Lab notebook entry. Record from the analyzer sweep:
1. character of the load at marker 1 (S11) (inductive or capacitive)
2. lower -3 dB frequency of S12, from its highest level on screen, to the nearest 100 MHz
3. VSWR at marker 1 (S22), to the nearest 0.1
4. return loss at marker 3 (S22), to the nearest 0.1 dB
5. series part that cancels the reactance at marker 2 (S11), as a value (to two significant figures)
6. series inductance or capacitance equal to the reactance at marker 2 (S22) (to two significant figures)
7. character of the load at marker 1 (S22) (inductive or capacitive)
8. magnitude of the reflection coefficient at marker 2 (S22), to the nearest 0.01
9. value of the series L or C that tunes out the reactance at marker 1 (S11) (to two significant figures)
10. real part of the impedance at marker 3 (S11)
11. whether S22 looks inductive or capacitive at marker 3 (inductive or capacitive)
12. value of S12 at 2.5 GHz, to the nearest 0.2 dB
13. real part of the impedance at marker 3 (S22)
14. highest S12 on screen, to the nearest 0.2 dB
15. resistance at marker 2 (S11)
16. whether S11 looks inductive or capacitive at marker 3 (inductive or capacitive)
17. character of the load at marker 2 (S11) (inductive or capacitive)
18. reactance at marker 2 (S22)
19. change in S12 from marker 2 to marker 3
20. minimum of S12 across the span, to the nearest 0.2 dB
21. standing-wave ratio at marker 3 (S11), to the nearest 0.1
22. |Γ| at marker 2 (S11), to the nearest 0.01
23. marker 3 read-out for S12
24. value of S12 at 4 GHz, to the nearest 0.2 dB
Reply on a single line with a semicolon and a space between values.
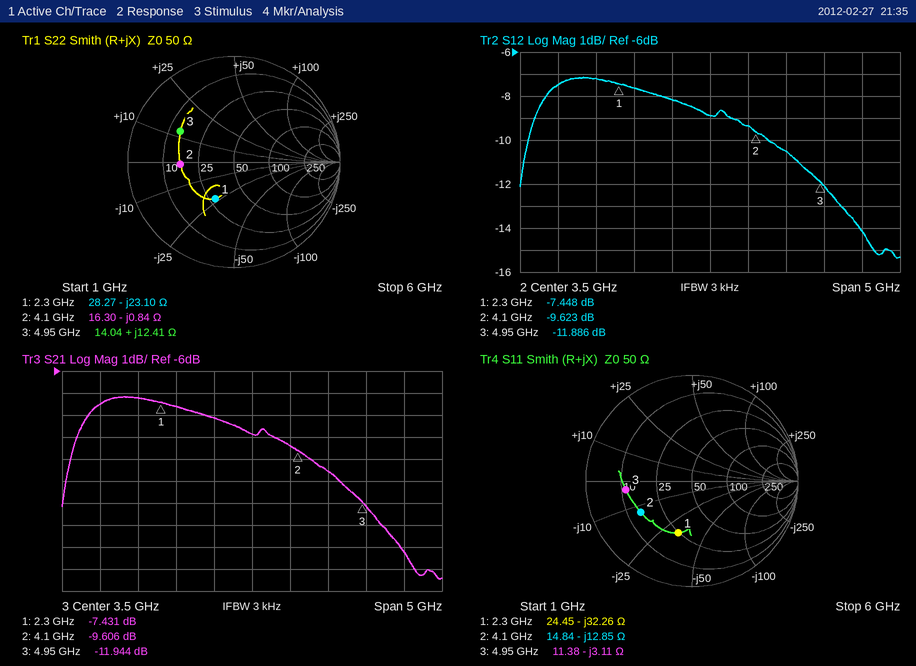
capacitive; 1.1 GHz; 2.3; 4.7 dB; 500 pH; 46 pF; capacitive; 0.51; 2.2 nH; 11.38 Ω; inductive; -7.6 dB; 14.04 Ω; -7.2 dB; 14.84 Ω; capacitive; capacitive; -0.84 Ω; -2.263 dB; -15.4 dB; 4.4; 0.57; -11.886 dB; -9.4 dB
